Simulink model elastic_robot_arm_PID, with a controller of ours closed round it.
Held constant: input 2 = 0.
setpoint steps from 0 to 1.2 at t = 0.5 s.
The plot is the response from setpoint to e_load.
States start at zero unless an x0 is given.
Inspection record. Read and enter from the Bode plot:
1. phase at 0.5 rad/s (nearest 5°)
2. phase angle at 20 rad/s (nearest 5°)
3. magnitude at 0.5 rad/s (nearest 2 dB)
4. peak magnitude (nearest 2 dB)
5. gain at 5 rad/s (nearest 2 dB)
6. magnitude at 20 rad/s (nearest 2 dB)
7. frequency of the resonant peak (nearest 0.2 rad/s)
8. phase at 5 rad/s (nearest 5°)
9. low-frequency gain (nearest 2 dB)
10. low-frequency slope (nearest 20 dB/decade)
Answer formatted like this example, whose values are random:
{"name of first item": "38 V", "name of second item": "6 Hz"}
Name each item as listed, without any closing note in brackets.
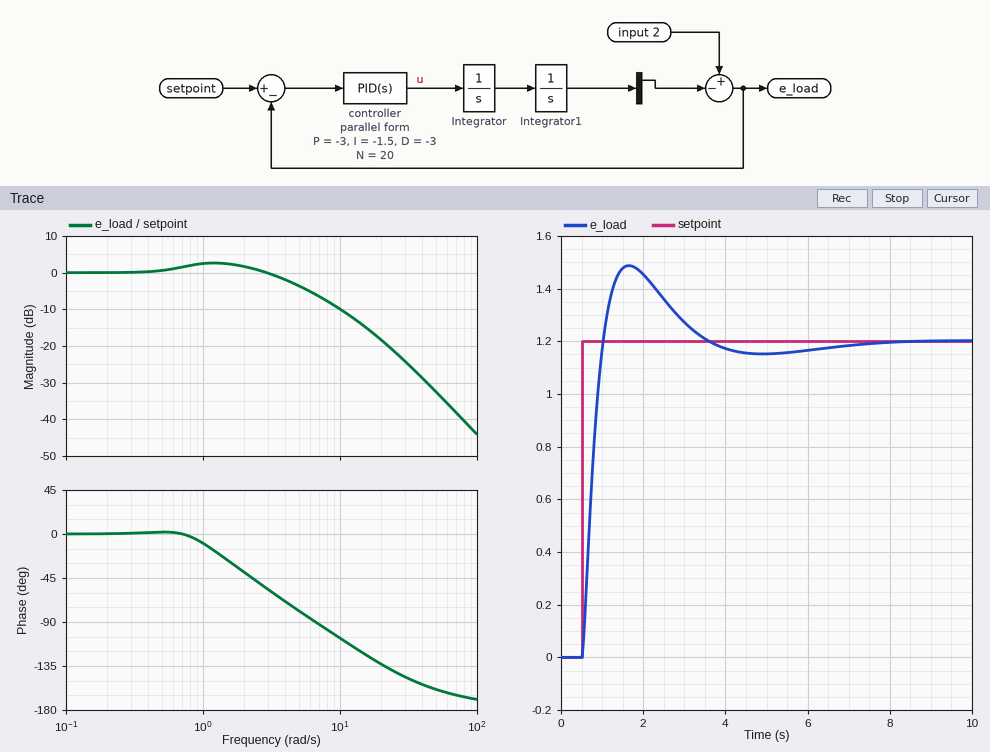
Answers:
{"phase at 0.5 rad/s": "0°", "phase angle at 20 rad/s": "-135°", "magnitude at 0.5 rad/s": "0 dB", "peak magnitude": "2 dB", "gain at 5 rad/s": "-4 dB", "magnitude at 20 rad/s": "-18 dB", "frequency of the resonant peak": "1.2 rad/s", "phase at 5 rad/s": "-80°", "low-frequency gain": "0 dB", "low-frequency slope": "0 dB/decade"}
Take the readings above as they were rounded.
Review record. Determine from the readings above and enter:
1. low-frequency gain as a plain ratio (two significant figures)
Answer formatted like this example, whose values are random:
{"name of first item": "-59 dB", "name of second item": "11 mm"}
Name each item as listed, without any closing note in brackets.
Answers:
{"low-frequency gain as a plain ratio": "1.0"}
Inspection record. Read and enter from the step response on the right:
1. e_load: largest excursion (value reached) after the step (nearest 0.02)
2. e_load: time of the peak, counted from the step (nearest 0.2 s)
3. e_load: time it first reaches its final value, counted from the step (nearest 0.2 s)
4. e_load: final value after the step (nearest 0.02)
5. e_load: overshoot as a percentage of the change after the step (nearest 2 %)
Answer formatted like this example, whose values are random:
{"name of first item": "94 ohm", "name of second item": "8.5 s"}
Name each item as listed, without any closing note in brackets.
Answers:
{"e_load: largest excursion (value reached) after the step": "1.48", "e_load: time of the peak, counted from the step": "1.2 s", "e_load: time it first reaches its final value, counted from the step": "0.6 s", "e_load: final value after the step": "1.20", "e_load: overshoot as a percentage of the change after the step": "24 %"}
